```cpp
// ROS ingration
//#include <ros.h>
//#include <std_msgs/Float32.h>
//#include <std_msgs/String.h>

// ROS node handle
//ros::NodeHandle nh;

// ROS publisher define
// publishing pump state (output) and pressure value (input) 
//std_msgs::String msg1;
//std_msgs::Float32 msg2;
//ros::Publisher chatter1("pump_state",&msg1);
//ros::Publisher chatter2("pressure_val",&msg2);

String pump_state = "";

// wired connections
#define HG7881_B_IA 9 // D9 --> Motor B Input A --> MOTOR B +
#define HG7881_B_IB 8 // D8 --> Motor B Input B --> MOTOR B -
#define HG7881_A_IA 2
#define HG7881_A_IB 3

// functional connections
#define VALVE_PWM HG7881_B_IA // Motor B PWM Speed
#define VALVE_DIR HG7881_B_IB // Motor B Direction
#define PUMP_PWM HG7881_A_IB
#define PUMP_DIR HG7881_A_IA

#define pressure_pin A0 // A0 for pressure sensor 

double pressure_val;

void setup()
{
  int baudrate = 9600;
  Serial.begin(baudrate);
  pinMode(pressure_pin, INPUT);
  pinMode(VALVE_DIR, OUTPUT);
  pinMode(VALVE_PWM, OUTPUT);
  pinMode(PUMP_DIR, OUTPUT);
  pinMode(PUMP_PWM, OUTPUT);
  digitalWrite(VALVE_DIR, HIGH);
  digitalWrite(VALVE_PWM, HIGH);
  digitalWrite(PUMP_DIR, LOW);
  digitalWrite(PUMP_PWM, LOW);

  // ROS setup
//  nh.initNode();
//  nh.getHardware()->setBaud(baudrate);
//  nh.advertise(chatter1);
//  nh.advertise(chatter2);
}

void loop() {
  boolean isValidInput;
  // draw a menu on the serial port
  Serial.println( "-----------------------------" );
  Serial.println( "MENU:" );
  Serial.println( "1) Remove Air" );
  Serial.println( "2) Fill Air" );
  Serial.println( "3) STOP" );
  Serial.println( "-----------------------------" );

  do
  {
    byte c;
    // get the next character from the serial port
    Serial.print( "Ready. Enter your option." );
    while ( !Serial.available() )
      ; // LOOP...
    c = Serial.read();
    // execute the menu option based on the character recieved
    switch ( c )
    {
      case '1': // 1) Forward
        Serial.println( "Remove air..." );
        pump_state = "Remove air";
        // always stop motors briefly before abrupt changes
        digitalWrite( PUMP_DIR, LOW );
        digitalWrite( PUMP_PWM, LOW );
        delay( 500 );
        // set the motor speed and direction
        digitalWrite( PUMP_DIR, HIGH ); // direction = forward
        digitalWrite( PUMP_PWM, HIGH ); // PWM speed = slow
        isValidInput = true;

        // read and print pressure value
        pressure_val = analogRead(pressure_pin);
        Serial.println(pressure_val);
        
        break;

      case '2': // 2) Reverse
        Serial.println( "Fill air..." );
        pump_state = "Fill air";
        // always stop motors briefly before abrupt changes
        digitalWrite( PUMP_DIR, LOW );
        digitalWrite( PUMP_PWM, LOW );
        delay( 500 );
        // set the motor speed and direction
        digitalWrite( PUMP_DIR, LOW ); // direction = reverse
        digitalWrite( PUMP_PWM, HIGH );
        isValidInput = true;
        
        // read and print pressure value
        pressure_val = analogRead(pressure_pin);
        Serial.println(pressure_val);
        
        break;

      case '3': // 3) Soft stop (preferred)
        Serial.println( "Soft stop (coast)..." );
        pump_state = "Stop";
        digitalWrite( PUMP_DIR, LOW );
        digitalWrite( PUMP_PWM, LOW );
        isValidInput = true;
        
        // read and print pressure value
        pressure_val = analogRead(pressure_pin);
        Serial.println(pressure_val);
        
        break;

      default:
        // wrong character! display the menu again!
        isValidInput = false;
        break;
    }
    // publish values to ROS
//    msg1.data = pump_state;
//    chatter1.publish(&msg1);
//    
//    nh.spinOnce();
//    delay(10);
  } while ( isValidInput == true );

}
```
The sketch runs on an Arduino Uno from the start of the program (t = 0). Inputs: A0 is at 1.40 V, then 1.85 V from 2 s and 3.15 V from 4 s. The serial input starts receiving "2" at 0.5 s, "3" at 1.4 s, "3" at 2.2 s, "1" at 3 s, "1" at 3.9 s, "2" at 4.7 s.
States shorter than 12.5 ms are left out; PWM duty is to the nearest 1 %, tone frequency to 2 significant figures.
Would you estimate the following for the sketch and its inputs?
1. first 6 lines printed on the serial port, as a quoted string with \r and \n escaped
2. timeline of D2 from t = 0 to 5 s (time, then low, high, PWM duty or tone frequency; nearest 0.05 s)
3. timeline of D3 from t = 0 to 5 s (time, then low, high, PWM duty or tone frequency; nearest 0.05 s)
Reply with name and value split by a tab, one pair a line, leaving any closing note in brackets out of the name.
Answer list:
first 6 lines printed on the serial port, as a quoted string with \r and \n escaped	"-----------------------------\r\nMENU:\r\n1) Remove Air\r\n2) Fill Air\r\n3) STOP\r\n-----------------------------\r\n"
timeline of D2 from t = 0 to 5 s	0 s low; 3.5 s high; 3.9 s low; 4.4 s high; 4.7 s low
timeline of D3 from t = 0 to 5 s	0 s low; 1 s high; 1.4 s low; 3.5 s high; 3.9 s low; 4.4 s high; 4.7 s low
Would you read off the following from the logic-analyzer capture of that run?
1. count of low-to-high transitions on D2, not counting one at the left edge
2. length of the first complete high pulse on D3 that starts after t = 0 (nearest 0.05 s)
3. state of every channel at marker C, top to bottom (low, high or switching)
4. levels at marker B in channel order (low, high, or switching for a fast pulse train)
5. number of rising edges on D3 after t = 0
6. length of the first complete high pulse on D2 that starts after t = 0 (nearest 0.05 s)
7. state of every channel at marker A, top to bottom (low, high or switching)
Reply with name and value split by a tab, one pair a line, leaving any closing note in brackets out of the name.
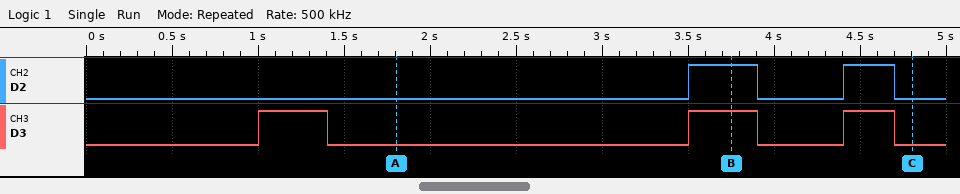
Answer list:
count of low-to-high transitions on D2, not counting one at the left edge	2
length of the first complete high pulse on D3 that starts after t = 0	0.40 s
state of every channel at marker C, top to bottom	D2 low, D3 low
levels at marker B in channel order	D2 high, D3 high
number of rising edges on D3 after t = 0	3
length of the first complete high pulse on D2 that starts after t = 0	0.40 s
state of every channel at marker A, top to bottom	D2 low, D3 low
